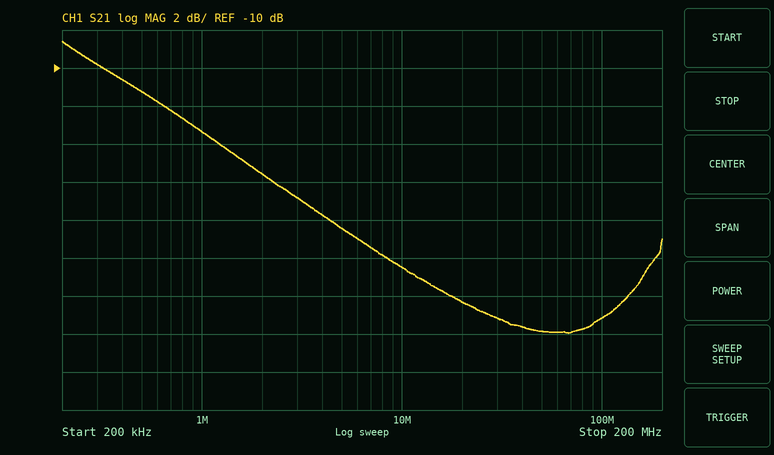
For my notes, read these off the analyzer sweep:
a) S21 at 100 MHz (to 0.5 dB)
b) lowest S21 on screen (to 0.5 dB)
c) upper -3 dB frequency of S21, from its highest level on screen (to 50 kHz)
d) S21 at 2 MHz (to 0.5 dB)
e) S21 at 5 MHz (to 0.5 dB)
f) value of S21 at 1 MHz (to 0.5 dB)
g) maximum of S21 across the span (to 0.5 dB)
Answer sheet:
-23.0 dB
-24.0 dB
550 kHz
-15.5 dB
-18.5 dB
-13.5 dB
-8.5 dB
